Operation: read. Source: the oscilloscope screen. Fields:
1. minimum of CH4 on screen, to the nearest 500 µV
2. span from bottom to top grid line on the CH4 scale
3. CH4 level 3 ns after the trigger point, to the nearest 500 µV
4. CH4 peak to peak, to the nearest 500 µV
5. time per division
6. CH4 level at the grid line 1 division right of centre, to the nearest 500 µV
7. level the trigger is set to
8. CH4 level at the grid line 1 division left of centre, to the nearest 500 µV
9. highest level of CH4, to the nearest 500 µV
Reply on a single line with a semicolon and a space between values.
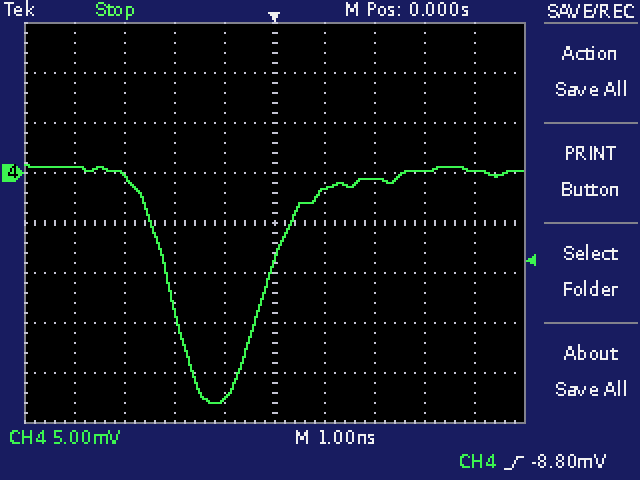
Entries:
-23.0 mV; 40 mV; 0.0 mV; 24.0 mV; 1 ns; -1.5 mV; -8.80 mV; -22.5 mV; 1.0 mV
